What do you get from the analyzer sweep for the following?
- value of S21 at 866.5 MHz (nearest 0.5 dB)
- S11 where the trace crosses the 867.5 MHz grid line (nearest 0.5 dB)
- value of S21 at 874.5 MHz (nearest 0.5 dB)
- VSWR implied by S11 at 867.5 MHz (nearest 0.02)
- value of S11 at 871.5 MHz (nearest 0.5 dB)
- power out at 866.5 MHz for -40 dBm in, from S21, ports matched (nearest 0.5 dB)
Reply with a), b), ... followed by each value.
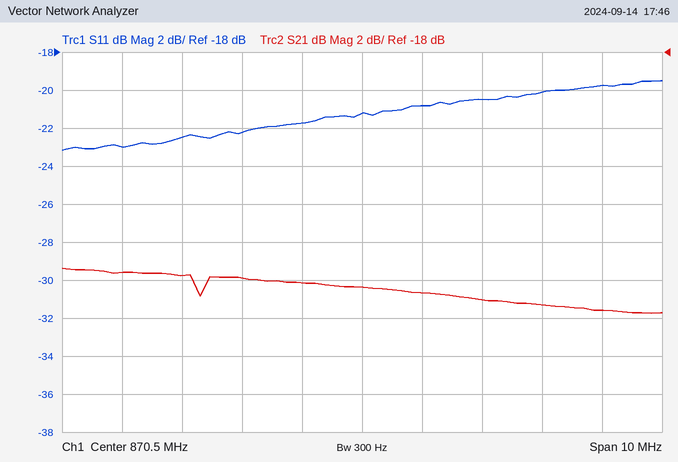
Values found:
a) -29.5 dB
b) -22.5 dB
c) -31.5 dB
d) 1.16
e) -21.0 dB
f) -69.5 dBm
